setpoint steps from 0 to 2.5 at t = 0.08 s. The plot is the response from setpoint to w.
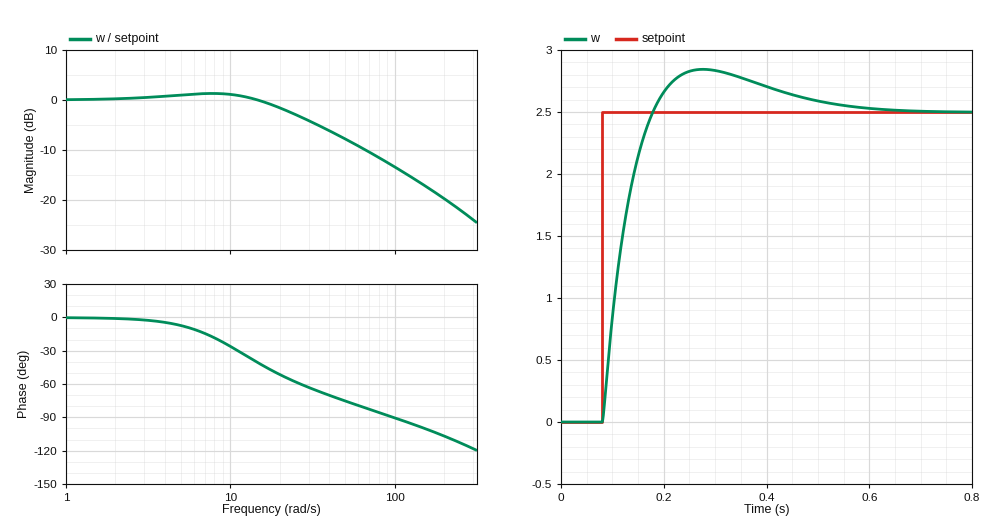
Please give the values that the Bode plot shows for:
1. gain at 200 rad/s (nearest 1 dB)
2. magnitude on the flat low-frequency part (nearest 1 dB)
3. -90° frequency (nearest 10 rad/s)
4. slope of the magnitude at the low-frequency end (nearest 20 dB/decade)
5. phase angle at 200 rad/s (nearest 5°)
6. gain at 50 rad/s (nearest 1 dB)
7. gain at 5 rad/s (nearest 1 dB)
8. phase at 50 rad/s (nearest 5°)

-20 dB
0 dB
100 rad/s
0 dB/decade
-105°
-8 dB
1 dB
-75°
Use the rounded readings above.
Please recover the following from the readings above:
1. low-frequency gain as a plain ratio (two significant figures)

1.0
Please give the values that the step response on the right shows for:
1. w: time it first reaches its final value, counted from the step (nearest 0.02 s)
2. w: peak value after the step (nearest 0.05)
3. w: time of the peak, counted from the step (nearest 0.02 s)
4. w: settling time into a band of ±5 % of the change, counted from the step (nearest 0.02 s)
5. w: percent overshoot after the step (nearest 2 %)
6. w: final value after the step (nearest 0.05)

0.10 s
2.85
0.20 s
0.38 s
14 %
2.50
